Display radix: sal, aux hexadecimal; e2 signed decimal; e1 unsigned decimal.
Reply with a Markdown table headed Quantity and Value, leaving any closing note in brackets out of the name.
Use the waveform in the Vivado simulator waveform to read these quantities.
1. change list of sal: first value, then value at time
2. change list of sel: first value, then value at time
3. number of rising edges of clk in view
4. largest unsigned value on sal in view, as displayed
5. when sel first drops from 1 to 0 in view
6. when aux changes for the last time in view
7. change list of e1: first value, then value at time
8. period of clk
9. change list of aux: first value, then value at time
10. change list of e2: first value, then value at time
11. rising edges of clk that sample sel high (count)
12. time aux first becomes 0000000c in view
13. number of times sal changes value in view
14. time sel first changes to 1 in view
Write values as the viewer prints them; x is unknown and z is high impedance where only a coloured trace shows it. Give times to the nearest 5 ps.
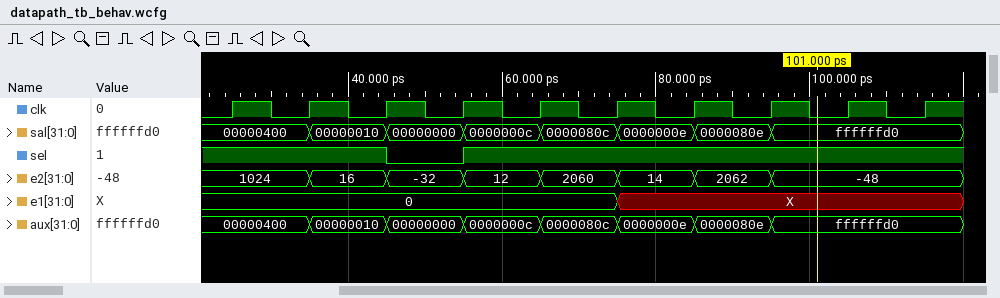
| Quantity | Value |
|---|---|
| change list of sal: first value, then value at time | 00000400, 00000010 at 35 ps, 00000000 at 45 ps, 0000000c at 55 ps, 0000080c at 65 ps, 0000000e at 75 ps, 0000080e at 85 ps, ffffffd0 at 95 ps |
| change list of sel: first value, then value at time | 1, 0 at 45 ps, 1 at 55 ps |
| number of rising edges of clk in view | 10 |
| largest unsigned value on sal in view, as displayed | ffffffd0 |
| when sel first drops from 1 to 0 in view | 45 ps |
| when aux changes for the last time in view | 95 ps |
| change list of e1: first value, then value at time | 0, X at 75 ps |
| period of clk | 10 ps |
| change list of aux: first value, then value at time | 00000400, 00000010 at 35 ps, 00000000 at 45 ps, 0000000c at 55 ps, 0000080c at 65 ps, 0000000e at 75 ps, 0000080e at 85 ps, ffffffd0 at 95 ps |
| change list of e2: first value, then value at time | 1024, 16 at 35 ps, -32 at 45 ps, 12 at 55 ps, 2060 at 65 ps, 14 at 75 ps, 2062 at 85 ps, -48 at 95 ps |
| rising edges of clk that sample sel high | 9 |
| time aux first becomes 0000000c in view | 55 ps |
| number of times sal changes value in view | 7 |
| time sel first changes to 1 in view | 55 ps |
